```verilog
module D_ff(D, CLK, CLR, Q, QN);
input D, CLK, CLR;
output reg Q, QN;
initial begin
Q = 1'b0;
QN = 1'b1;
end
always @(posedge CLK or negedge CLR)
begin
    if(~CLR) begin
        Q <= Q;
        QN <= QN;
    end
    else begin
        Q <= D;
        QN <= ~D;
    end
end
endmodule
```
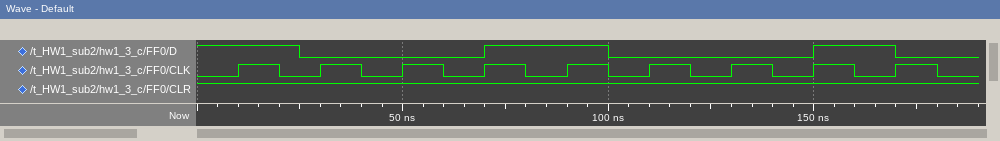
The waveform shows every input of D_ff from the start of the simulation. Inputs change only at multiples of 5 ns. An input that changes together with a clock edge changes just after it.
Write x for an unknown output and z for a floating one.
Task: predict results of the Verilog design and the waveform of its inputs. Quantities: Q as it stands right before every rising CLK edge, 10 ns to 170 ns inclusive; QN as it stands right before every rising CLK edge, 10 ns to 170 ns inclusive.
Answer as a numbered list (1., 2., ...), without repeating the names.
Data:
1. 0 1 0 0 0 1 0 0 0
2. 1 0 1 1 1 0 1 1 1
